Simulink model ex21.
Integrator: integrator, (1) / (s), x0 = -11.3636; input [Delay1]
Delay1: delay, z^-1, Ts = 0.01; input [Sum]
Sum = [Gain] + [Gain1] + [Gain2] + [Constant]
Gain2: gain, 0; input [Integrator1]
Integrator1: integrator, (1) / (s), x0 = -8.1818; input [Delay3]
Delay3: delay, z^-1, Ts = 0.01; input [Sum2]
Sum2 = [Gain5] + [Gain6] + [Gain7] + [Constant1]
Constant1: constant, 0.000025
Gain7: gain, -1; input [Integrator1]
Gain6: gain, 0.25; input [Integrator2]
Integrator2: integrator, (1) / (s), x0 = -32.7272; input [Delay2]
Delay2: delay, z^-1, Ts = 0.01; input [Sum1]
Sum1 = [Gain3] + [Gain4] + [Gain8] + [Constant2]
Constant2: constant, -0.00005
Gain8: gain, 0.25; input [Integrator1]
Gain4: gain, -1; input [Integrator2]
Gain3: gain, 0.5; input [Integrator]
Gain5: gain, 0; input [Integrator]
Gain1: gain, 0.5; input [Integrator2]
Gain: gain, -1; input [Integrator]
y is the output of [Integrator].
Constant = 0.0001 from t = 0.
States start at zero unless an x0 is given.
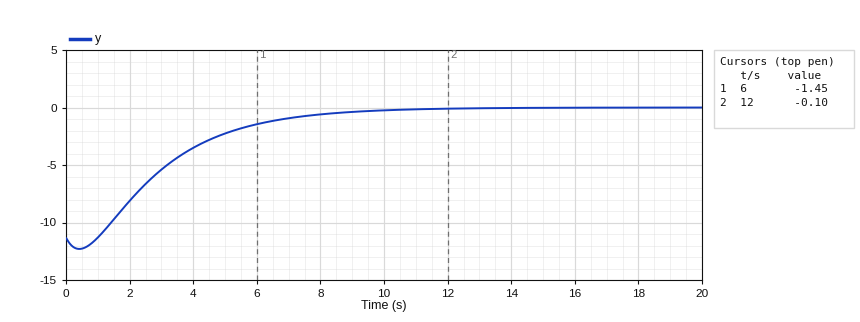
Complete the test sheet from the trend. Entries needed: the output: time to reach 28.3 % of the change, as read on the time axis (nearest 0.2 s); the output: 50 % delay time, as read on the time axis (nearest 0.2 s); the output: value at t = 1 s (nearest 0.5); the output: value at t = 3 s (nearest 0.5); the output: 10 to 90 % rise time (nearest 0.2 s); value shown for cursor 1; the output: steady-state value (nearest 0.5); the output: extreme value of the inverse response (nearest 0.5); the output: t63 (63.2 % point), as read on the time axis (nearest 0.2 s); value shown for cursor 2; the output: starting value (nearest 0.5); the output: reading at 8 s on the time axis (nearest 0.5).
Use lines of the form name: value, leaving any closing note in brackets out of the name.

the output: time to reach 28.3 % of the change, as read on the time axis: 2.0 s
the output: 50 % delay time, as read on the time axis: 2.8 s
the output: value at t = 1 s: -11.5
the output: value at t = 3 s: -5.5
the output: 10 to 90 % rise time: 5.2 s
value shown for cursor 1: -1.45
the output: steady-state value: 0.0
the output: extreme value of the inverse response: -12.5
the output: t63 (63.2 % point), as read on the time axis: 3.6 s
value shown for cursor 2: -0.10
the output: starting value: -11.5
the output: reading at 8 s on the time axis: -0.5
